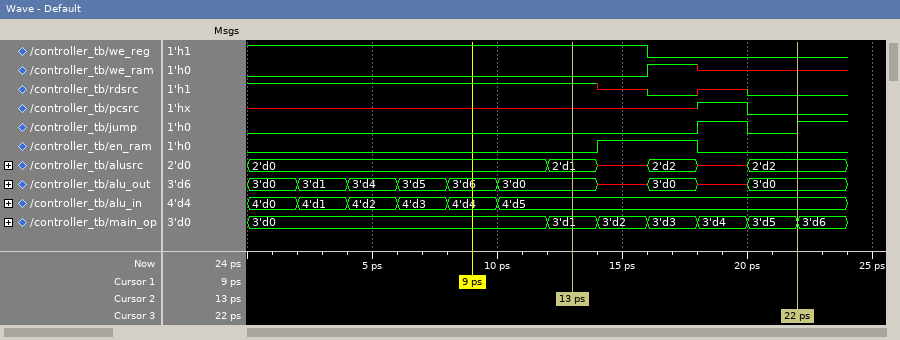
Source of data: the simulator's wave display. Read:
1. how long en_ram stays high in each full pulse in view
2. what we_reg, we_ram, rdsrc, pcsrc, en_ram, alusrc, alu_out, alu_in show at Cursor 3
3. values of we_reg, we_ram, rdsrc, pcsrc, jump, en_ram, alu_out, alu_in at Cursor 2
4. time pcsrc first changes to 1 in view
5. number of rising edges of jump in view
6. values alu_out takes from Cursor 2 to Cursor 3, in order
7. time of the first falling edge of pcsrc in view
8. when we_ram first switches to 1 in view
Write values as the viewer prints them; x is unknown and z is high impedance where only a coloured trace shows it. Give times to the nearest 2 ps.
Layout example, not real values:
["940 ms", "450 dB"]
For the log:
["4 ps", "we_reg=0, we_ram=x, rdsrc=0, pcsrc=0, en_ram=0, alusrc=2'd2, alu_out=3'd0, alu_in=4'd5", "we_reg=1, we_ram=0, rdsrc=1, pcsrc=x, jump=0, en_ram=0, alu_out=3'd0, alu_in=4'd5", "18 ps", "2", "3'd0, x, 3'd0, x, 3'd0", "20 ps", "16 ps"]
